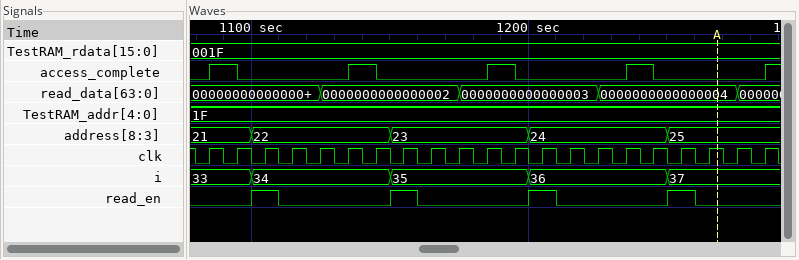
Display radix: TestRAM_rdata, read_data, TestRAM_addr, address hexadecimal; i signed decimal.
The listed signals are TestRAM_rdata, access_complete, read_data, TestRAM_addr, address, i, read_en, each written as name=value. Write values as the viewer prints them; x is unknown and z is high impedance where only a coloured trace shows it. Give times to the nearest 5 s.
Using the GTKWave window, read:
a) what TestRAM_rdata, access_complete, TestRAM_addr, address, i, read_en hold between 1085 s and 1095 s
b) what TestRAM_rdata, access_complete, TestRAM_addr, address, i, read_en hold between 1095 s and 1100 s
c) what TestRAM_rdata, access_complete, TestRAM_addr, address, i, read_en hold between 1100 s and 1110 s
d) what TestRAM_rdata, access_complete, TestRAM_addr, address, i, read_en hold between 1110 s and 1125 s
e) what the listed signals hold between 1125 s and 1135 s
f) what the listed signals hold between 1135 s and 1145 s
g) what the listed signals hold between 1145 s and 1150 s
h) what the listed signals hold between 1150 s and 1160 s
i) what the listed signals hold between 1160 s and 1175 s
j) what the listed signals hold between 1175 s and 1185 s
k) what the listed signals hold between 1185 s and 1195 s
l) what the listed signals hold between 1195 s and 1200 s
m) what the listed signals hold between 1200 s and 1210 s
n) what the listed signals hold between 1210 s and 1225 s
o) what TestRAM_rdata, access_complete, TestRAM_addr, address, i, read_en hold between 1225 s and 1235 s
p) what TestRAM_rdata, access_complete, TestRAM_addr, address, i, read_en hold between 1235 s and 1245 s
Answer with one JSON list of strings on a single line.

["TestRAM_rdata=001F, access_complete=1, TestRAM_addr=1F, address=21, i=33, read_en=0", "TestRAM_rdata=001F, access_complete=0, TestRAM_addr=1F, address=21, i=33, read_en=0", "TestRAM_rdata=001F, access_complete=0, TestRAM_addr=1F, address=22, i=34, read_en=1", "TestRAM_rdata=001F, access_complete=0, TestRAM_addr=1F, address=22, i=34, read_en=0", "TestRAM_rdata=001F, access_complete=0, read_data=0000000000000002, TestRAM_addr=1F, address=22, i=34, read_en=0", "TestRAM_rdata=001F, access_complete=1, read_data=0000000000000002, TestRAM_addr=1F, address=22, i=34, read_en=0", "TestRAM_rdata=001F, access_complete=0, read_data=0000000000000002, TestRAM_addr=1F, address=22, i=34, read_en=0", "TestRAM_rdata=001F, access_complete=0, read_data=0000000000000002, TestRAM_addr=1F, address=23, i=35, read_en=1", "TestRAM_rdata=001F, access_complete=0, read_data=0000000000000002, TestRAM_addr=1F, address=23, i=35, read_en=0", "TestRAM_rdata=001F, access_complete=0, read_data=0000000000000003, TestRAM_addr=1F, address=23, i=35, read_en=0", "TestRAM_rdata=001F, access_complete=1, read_data=0000000000000003, TestRAM_addr=1F, address=23, i=35, read_en=0", "TestRAM_rdata=001F, access_complete=0, read_data=0000000000000003, TestRAM_addr=1F, address=23, i=35, read_en=0", "TestRAM_rdata=001F, access_complete=0, read_data=0000000000000003, TestRAM_addr=1F, address=24, i=36, read_en=1", "TestRAM_rdata=001F, access_complete=0, read_data=0000000000000003, TestRAM_addr=1F, address=24, i=36, read_en=0", "TestRAM_rdata=001F, access_complete=0, TestRAM_addr=1F, address=24, i=36, read_en=0", "TestRAM_rdata=001F, access_complete=1, TestRAM_addr=1F, address=24, i=36, read_en=0"]
